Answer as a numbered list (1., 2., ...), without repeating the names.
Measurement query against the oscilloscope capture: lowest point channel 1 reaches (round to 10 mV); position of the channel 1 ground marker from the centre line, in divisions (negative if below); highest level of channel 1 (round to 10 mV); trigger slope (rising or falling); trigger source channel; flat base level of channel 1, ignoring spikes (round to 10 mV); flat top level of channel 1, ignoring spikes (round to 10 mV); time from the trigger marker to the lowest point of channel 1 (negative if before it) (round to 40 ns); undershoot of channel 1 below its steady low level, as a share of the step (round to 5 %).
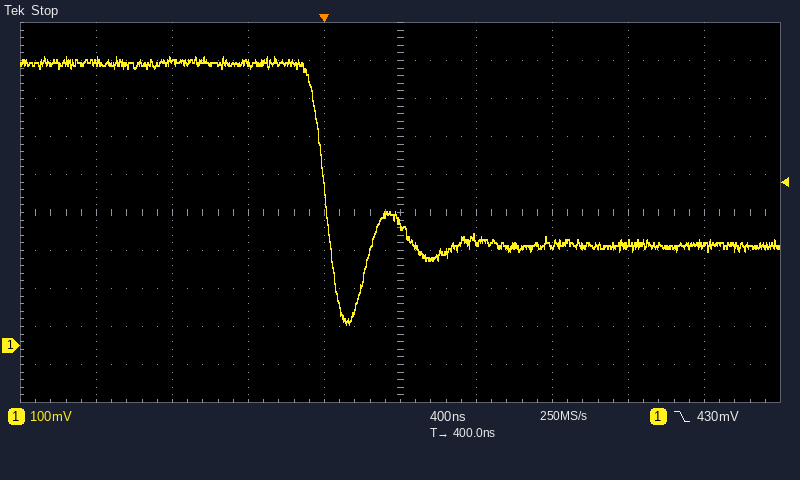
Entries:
1. 60 mV
2. -3.5 div
3. 760 mV
4. falling
5. channel 1
6. 260 mV
7. 740 mV
8. +120 ns
9. 45 %
